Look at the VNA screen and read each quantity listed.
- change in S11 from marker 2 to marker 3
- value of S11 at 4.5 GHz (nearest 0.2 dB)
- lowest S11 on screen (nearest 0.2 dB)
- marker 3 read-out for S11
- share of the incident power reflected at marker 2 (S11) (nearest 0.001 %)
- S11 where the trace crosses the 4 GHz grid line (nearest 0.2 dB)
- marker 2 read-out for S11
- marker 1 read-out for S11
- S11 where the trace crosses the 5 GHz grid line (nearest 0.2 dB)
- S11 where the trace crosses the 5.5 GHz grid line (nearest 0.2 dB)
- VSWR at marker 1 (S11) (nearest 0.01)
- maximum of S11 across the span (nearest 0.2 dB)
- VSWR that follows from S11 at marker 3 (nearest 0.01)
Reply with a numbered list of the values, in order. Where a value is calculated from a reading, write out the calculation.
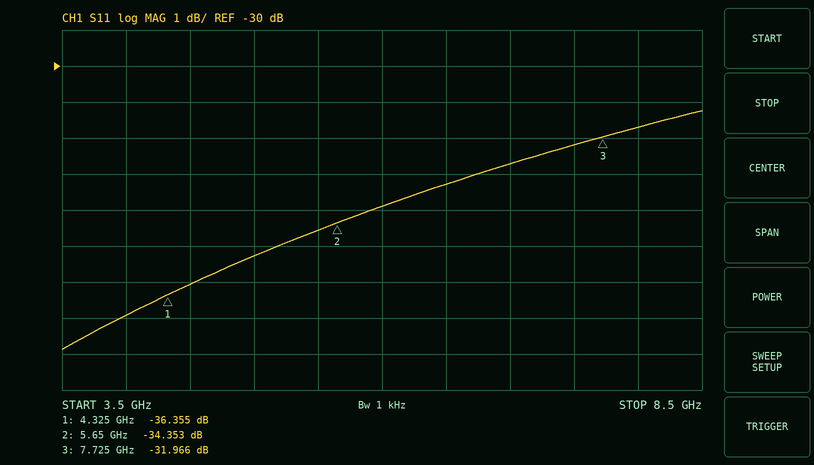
1. -31.966 − (-34.353) = 2.387 dB
2. -36.0 dB
3. -37.8 dB
4. -31.966 dB
5. 10^(-34.353/10) ≈ 0.037 %
6. -37.0 dB
7. -34.353 dB
8. -36.355 dB
9. -35.2 dB
10. -34.6 dB
11. (1 + 0.0152)/(1 − 0.0152) ≈ 1.03
12. -31.2 dB
13. (1 + 0.0252)/(1 − 0.0252) ≈ 1.05
